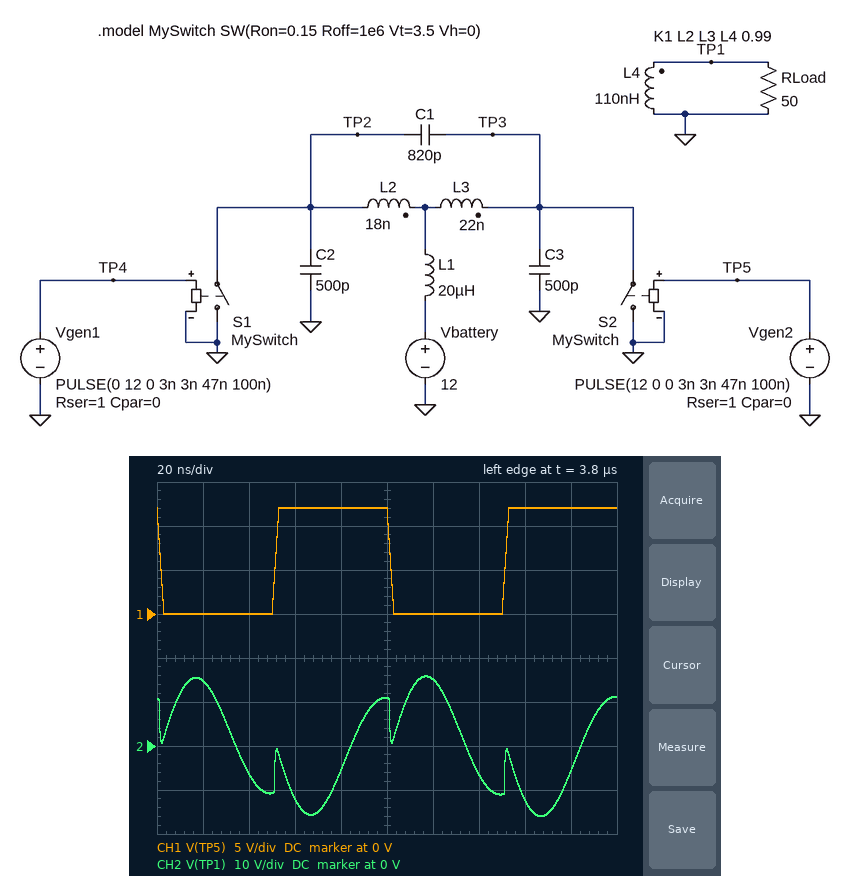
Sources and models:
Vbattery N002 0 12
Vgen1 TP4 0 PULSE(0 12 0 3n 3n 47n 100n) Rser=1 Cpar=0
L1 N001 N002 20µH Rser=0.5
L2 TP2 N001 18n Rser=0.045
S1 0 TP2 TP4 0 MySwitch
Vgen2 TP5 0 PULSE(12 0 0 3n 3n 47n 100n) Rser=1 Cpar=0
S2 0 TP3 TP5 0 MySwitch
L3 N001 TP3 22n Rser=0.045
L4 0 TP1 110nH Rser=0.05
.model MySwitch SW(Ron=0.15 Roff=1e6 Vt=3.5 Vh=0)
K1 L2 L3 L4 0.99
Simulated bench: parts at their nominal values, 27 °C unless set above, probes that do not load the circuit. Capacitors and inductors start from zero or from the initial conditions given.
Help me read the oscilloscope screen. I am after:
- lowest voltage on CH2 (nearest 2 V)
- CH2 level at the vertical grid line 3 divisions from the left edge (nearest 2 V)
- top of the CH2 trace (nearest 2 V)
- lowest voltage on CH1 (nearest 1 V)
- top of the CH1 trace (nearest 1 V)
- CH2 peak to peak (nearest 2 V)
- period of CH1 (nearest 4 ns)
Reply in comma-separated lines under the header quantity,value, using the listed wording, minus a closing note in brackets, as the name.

quantity,value
lowest voltage on CH2,-16 V
CH2 level at the vertical grid line 3 divisions from the left edge,-12 V
top of the CH2 trace,16 V
lowest voltage on CH1,0 V
top of the CH1 trace,12 V
CH2 peak to peak,32 V
period of CH1,100 ns
